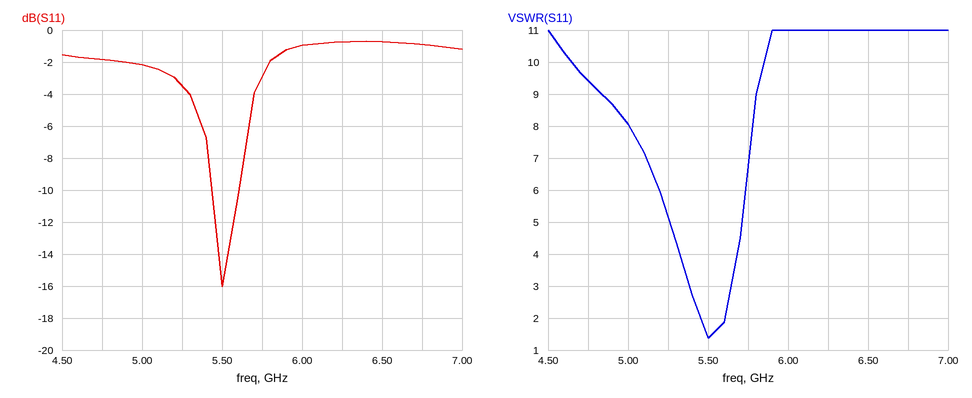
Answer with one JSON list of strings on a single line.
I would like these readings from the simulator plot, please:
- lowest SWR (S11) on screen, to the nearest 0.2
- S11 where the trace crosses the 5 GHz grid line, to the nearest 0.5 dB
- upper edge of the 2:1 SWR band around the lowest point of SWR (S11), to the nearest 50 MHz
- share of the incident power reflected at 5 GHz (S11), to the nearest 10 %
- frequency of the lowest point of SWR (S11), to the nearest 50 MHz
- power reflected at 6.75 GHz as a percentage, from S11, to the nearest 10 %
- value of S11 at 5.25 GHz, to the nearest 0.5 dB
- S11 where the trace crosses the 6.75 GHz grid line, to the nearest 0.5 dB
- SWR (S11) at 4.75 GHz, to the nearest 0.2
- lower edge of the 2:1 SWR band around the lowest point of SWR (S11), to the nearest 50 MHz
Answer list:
["1.4", "-2.0 dB", "5.60 GHz", "60 %", "5.50 GHz", "80 %", "-3.5 dB", "-1.0 dB", "9.4", "5.45 GHz"]
